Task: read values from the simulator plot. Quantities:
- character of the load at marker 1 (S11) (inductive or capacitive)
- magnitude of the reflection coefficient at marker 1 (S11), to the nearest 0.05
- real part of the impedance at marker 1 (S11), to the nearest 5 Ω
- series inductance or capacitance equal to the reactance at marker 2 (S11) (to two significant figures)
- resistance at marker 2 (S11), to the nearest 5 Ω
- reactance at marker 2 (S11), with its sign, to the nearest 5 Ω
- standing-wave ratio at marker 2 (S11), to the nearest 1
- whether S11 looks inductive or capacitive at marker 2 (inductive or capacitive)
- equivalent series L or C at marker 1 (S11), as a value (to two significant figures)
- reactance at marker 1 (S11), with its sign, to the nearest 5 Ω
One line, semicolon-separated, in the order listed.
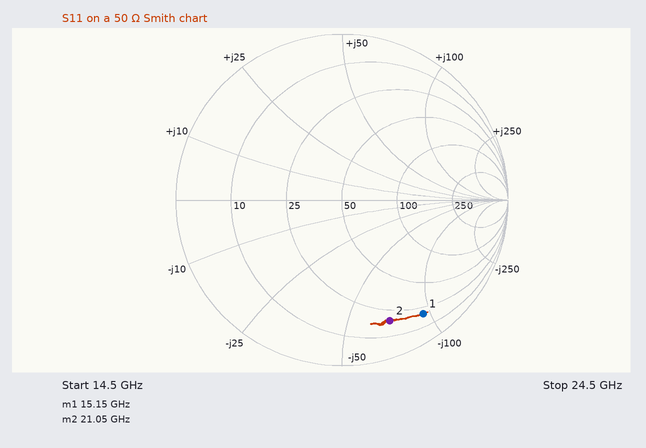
capacitive; 0.85; 20 Ω; 110 fF; 20 Ω; -70 Ω; 8; capacitive; 110 fF; -95 Ω
